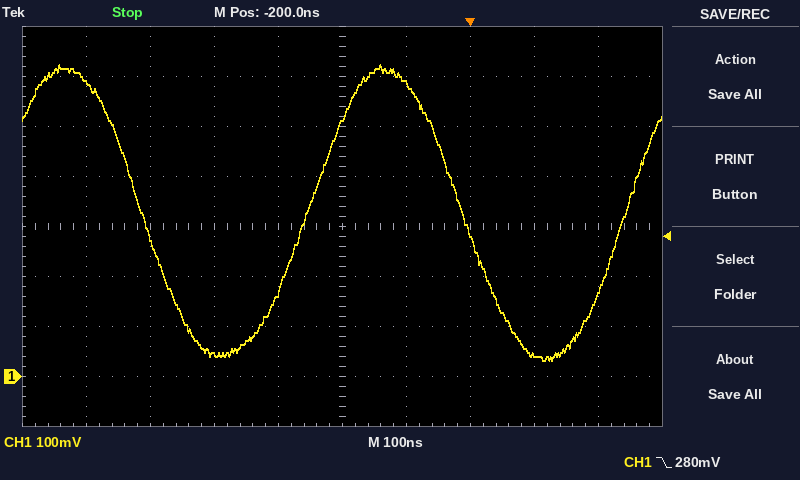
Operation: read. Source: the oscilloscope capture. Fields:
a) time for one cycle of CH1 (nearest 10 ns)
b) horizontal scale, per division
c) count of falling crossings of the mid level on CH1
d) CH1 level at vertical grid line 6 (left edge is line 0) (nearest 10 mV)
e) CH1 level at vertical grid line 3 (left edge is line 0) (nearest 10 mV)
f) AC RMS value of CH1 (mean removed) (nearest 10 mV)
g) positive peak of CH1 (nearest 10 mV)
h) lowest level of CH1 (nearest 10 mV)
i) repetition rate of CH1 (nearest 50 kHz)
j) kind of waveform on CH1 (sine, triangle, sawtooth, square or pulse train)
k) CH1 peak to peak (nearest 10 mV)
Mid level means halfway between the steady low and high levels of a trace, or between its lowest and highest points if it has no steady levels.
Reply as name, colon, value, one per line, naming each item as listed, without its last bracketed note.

time for one cycle of CH1: 500 ns
horizontal scale, per division: 100 ns
count of falling crossings of the mid level on CH1: 2
CH1 level at vertical grid line 6 (left edge is line 0): 580 mV
CH1 level at vertical grid line 3 (left edge is line 0): 40 mV
AC RMS value of CH1 (mean removed): 210 mV
positive peak of CH1: 620 mV
lowest level of CH1: 30 mV
repetition rate of CH1: 2.00 MHz
kind of waveform on CH1: sine
CH1 peak to peak: 590 mV
